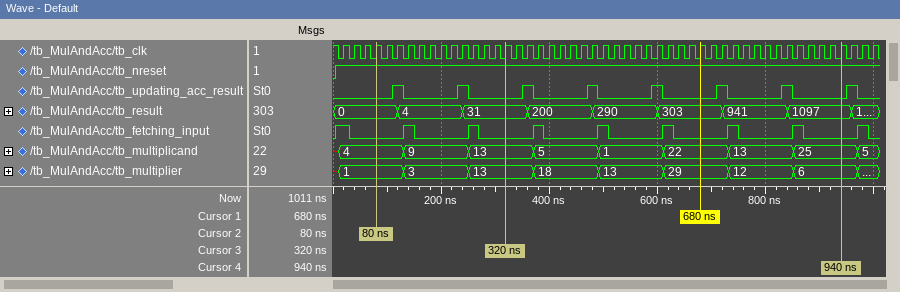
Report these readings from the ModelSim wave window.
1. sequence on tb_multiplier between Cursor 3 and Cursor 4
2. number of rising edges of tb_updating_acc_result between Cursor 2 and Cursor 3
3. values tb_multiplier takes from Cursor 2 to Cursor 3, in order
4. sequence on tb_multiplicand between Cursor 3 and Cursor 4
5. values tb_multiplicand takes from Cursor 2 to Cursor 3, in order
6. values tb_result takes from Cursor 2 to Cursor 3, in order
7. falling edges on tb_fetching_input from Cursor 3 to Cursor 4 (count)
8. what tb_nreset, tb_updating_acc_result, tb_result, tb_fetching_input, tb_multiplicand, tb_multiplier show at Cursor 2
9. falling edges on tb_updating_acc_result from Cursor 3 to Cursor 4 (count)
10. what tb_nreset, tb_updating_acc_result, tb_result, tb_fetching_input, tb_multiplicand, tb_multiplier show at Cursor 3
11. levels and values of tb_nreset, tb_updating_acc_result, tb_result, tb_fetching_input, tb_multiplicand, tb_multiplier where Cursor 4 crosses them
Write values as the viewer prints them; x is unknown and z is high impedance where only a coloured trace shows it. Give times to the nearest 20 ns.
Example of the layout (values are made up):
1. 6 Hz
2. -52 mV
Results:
1. 13, 18, 13, 29, 12, 6
2. 2
3. 1, 3, 13
4. 13, 5, 1, 22, 13, 25
5. 4, 9, 13
6. 0, 4, 31
7. 5
8. tb_nreset=1, tb_updating_acc_result=0, tb_result=0, tb_fetching_input=0, tb_multiplicand=4, tb_multiplier=1
9. 5
10. tb_nreset=1, tb_updating_acc_result=0, tb_result=31, tb_fetching_input=0, tb_multiplicand=13, tb_multiplier=13
11. tb_nreset=1, tb_updating_acc_result=0, tb_result=1097, tb_fetching_input=0, tb_multiplicand=25, tb_multiplier=6
